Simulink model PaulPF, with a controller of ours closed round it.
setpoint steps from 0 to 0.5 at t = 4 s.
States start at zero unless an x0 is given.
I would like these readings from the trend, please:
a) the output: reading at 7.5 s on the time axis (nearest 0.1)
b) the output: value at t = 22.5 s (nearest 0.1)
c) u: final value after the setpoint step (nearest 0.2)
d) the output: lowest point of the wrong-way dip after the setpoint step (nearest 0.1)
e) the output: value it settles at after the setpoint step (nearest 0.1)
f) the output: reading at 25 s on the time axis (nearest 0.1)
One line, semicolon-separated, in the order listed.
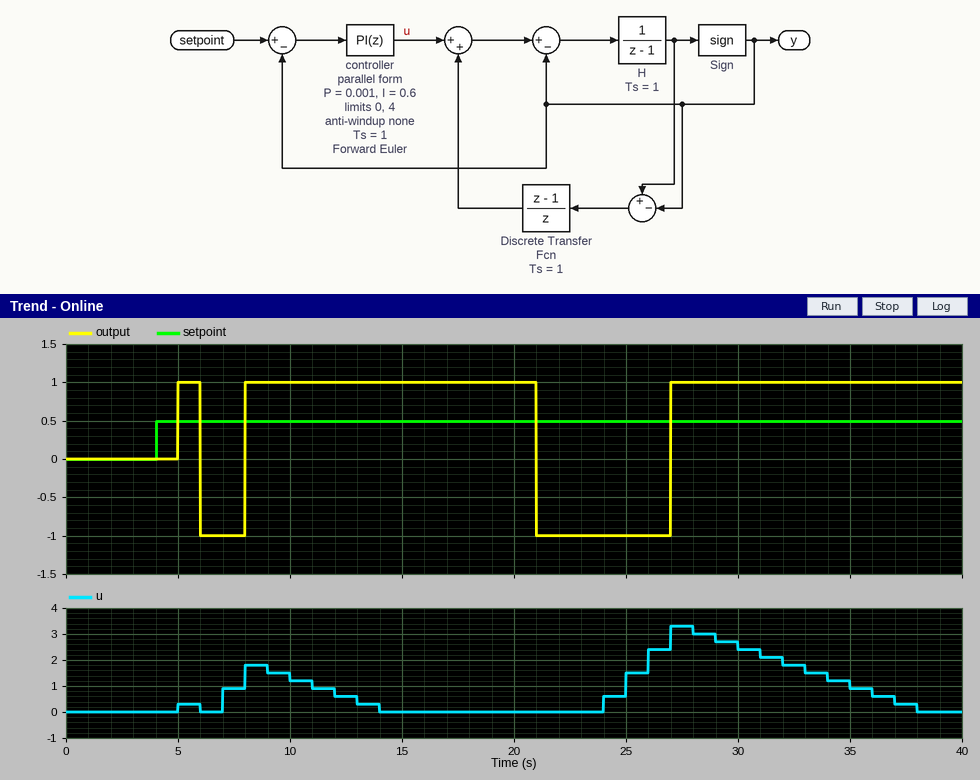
-1.0; -1.0; 0.0; -1.0; 1.0; -1.0
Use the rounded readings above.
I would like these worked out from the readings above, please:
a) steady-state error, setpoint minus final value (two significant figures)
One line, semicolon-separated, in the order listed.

-0.50
